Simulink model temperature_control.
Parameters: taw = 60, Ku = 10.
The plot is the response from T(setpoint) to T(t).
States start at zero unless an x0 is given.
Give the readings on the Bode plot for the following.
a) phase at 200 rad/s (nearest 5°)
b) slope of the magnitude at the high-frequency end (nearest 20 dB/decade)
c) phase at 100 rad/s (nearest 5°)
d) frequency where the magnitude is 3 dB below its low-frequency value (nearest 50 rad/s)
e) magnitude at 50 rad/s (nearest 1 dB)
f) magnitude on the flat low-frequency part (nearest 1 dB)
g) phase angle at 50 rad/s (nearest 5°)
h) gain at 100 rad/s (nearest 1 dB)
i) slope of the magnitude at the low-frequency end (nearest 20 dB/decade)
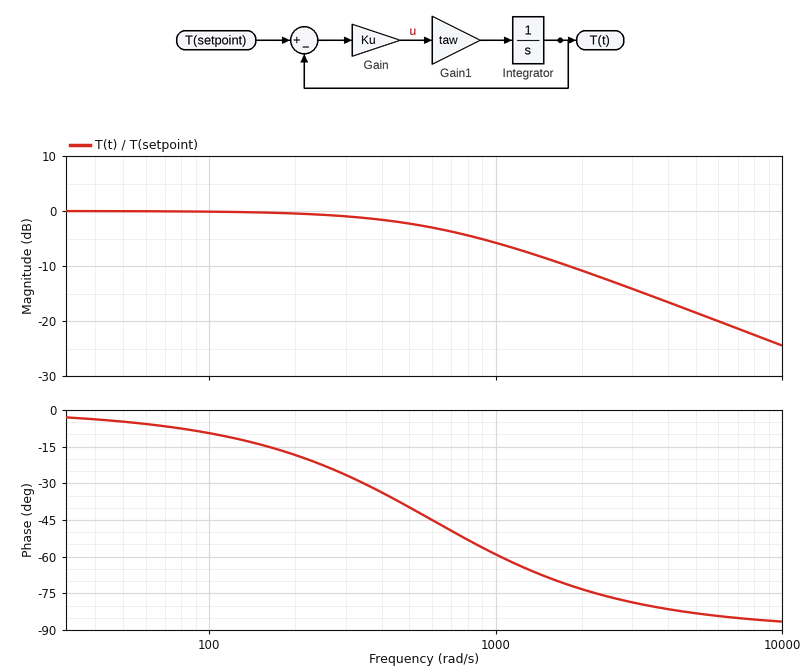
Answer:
-20°
-20 dB/decade
-10°
600 rad/s
0 dB
0 dB
-5°
0 dB
0 dB/decade
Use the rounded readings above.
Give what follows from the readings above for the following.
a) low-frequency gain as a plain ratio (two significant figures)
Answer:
1.0
